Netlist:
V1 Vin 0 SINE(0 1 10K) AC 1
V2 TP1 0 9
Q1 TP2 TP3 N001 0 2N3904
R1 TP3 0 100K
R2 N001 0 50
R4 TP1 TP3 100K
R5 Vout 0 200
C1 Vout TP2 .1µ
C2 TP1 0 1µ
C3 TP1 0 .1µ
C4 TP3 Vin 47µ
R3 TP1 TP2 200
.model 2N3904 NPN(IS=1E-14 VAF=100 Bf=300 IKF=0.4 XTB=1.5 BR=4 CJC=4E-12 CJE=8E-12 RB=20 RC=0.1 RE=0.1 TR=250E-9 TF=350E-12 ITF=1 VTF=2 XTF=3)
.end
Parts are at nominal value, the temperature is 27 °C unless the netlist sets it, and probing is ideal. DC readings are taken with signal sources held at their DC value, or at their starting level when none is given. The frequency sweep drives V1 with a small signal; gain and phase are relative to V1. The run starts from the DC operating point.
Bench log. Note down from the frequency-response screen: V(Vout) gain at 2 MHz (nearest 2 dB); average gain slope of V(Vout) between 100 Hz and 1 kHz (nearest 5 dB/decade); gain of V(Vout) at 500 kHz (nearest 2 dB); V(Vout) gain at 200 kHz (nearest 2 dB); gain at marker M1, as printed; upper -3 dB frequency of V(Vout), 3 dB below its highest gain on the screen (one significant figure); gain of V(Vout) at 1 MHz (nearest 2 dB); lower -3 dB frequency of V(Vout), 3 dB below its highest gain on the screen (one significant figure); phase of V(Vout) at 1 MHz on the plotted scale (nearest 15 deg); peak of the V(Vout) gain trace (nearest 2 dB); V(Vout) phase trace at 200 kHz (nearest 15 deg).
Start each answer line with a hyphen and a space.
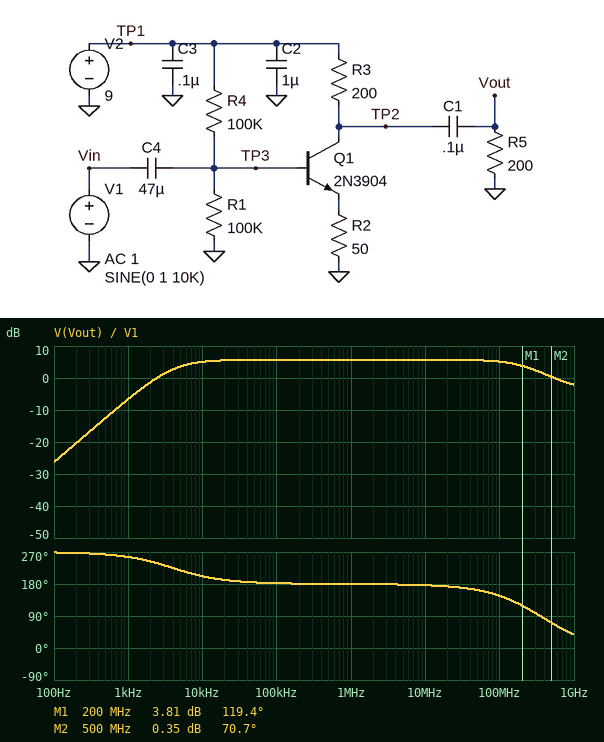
- 6 dB
- 20 dB/decade
- 6 dB
- 6 dB
- 3.81 dB
- 300 MHz
- 6 dB
- 4 kHz
- 180 deg
- 6 dB
- 180 deg
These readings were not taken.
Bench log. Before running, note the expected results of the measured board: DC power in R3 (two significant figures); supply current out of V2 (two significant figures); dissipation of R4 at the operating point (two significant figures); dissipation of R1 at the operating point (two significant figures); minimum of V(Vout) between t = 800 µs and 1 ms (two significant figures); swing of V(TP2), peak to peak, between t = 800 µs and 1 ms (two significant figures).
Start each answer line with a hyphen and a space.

- 60 mW
- 17 mA
- 550 µW
- 26 µW
- -1.8 V
- 4.4 V
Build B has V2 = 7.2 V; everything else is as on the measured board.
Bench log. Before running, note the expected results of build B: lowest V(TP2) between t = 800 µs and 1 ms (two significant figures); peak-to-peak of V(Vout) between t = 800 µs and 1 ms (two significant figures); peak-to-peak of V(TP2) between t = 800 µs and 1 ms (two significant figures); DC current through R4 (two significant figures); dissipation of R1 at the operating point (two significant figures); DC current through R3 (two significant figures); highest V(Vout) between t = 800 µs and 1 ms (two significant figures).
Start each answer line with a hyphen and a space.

- 2.2 V
- 3.3 V
- 4.1 V
- 58 µA
- 19 µW
- 13 mA
- 1.6 V
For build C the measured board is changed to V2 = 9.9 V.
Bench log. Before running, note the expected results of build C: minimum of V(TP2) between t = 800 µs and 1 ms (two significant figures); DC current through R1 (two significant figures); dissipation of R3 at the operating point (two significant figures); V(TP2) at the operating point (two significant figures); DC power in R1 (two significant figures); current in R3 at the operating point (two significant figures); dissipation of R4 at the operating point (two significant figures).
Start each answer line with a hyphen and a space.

- 3.7 V
- 17 µA
- 75 mW
- 6.0 V
- 29 µW
- 19 mA
- 670 µW
